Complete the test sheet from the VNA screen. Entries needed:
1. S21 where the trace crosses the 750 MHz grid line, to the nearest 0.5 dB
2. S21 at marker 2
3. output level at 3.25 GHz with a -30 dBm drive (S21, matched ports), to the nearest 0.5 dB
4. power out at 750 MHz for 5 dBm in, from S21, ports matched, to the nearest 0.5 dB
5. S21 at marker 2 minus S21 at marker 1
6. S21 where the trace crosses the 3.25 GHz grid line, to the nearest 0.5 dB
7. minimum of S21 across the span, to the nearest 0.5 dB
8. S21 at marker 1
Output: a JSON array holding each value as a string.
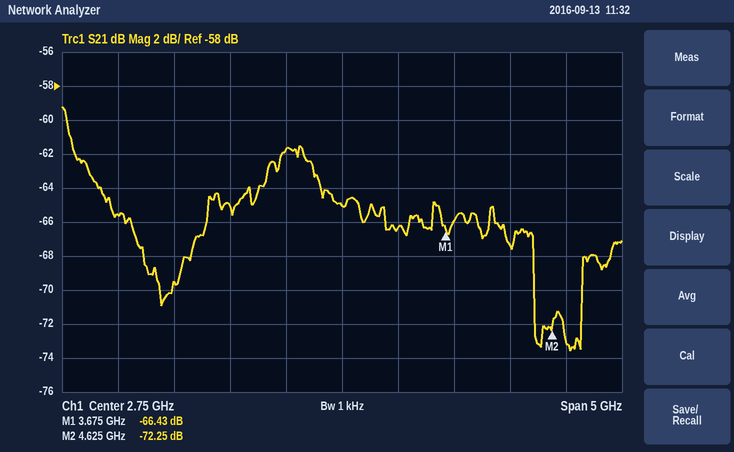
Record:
["-65.5 dB", "-72.25 dB", "-96.5 dBm", "-60.5 dBm", "-5.82 dB", "-66.5 dB", "-73.5 dB", "-66.43 dB"]
